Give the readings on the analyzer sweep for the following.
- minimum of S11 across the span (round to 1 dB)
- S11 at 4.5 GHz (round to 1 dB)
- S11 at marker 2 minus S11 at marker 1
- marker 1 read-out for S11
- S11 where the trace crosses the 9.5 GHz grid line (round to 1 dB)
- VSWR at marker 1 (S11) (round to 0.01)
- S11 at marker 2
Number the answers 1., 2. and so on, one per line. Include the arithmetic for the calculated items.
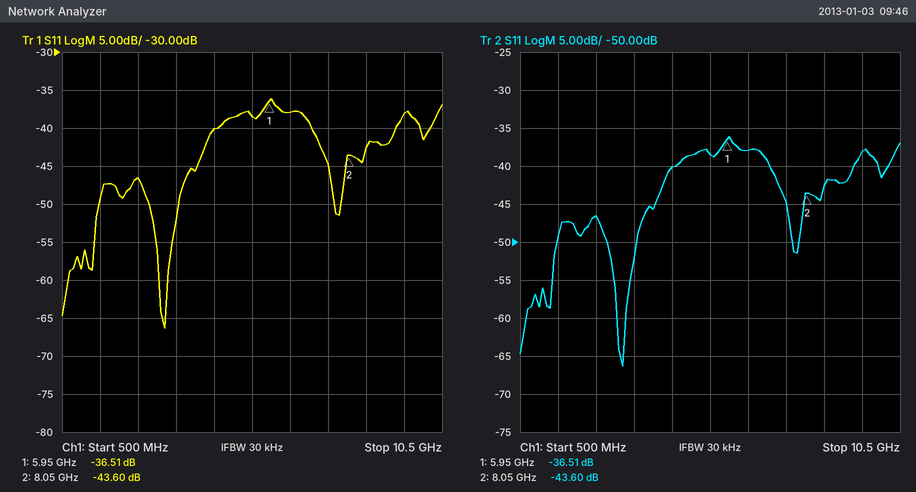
1. -66 dB
2. -40 dB
3. -43.6 − (-36.51) = -7.09 dB
4. -36.51 dB
5. -38 dB
6. (1 + 0.0149)/(1 − 0.0149) ≈ 1.03
7. -43.60 dB
